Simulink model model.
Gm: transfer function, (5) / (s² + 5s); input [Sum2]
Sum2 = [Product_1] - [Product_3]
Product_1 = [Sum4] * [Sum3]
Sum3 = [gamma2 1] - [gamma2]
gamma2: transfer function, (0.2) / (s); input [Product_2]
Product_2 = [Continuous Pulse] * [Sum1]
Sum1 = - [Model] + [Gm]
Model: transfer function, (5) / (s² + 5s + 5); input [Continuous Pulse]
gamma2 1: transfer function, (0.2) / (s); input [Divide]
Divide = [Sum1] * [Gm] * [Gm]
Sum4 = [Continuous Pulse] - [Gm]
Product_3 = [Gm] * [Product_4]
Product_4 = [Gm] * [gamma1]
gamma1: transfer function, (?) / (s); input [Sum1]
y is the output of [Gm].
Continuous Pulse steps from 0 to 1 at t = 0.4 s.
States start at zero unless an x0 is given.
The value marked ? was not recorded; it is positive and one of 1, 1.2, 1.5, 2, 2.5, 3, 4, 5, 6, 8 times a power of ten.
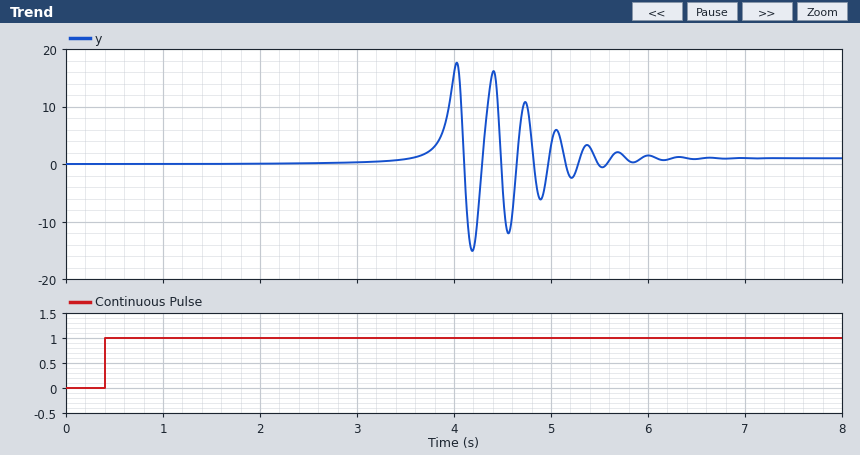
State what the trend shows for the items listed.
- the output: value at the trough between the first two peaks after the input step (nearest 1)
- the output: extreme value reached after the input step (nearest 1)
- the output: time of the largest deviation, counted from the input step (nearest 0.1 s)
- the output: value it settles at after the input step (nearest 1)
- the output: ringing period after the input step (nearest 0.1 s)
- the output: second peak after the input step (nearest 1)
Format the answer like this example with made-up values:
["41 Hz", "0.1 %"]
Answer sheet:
["-15", "18", "3.6 s", "1", "0.4 s", "16"]
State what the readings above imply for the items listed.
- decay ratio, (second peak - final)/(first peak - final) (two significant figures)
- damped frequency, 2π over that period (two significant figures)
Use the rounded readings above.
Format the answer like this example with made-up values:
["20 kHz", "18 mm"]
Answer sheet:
["0.88", "16 rad/s"]
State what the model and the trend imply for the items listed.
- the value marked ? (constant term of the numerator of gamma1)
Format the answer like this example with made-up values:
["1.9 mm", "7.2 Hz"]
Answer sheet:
["4"]
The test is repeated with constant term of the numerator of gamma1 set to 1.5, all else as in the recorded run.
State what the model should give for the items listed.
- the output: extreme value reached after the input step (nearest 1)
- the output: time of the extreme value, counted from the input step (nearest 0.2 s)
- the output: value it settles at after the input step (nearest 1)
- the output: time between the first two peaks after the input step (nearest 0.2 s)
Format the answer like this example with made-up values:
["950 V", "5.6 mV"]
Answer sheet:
["9", "4.4 s", "1", "0.6 s"]
